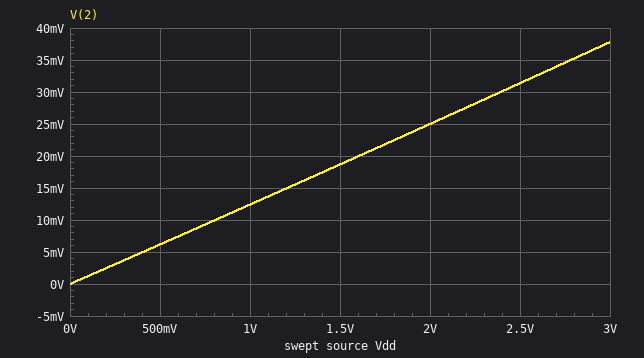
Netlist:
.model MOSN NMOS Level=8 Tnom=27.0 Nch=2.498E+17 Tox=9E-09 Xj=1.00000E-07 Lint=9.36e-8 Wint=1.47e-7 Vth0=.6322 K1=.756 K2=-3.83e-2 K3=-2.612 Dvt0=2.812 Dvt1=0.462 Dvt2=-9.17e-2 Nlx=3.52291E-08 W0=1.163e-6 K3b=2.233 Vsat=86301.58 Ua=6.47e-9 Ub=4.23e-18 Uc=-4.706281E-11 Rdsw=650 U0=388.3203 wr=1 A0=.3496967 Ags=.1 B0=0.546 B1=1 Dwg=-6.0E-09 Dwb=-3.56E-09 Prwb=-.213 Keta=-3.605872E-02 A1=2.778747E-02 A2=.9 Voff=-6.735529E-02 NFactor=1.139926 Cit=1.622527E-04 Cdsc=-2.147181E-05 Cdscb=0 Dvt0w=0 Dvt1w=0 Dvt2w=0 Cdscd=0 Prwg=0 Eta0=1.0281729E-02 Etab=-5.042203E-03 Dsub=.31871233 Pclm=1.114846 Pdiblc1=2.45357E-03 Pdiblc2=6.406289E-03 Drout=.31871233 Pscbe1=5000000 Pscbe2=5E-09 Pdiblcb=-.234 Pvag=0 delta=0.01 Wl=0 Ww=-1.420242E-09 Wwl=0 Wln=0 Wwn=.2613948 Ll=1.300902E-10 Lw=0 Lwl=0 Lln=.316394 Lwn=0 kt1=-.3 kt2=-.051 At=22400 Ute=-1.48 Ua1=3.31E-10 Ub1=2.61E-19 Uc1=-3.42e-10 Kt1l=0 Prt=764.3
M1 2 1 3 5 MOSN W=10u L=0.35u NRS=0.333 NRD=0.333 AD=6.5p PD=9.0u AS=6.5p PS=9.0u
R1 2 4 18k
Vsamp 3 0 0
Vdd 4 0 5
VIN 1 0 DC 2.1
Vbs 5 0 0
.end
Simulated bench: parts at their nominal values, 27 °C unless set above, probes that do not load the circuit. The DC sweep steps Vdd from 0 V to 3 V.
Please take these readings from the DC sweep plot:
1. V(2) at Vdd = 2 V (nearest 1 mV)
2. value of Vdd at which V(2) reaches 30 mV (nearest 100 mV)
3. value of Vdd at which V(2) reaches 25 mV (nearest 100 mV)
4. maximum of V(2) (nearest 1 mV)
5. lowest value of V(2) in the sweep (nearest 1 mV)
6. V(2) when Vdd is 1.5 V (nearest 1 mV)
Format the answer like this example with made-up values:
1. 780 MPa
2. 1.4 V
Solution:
1. 25 mV
2. 2.4 V
3. 2.0 V
4. 38 mV
5. 0 V
6. 19 mV
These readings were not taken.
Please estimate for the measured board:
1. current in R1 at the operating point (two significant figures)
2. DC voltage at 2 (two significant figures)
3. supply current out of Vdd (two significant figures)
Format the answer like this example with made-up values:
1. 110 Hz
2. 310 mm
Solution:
1. 270 µA
2. 64 mV
3. 270 µA
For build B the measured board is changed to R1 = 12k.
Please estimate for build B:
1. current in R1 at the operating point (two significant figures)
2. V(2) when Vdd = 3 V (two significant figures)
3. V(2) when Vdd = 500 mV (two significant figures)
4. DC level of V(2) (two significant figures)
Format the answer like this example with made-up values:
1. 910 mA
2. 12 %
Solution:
1. 410 µA
2. 57 mV
3. 9.2 mV
4. 97 mV
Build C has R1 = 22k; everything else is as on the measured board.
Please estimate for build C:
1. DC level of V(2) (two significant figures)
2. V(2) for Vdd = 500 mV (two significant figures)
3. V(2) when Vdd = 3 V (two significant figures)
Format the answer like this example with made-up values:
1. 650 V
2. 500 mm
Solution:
1. 52 mV
2. 5.1 mV
3. 31 mV
